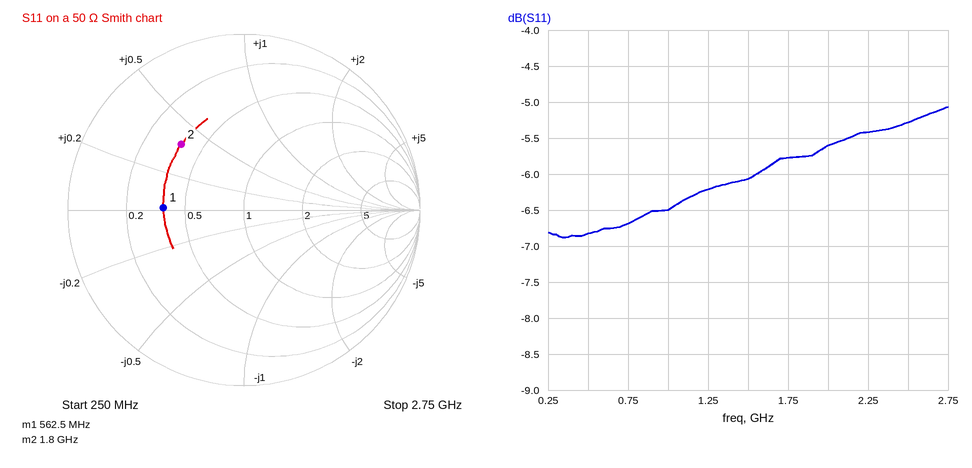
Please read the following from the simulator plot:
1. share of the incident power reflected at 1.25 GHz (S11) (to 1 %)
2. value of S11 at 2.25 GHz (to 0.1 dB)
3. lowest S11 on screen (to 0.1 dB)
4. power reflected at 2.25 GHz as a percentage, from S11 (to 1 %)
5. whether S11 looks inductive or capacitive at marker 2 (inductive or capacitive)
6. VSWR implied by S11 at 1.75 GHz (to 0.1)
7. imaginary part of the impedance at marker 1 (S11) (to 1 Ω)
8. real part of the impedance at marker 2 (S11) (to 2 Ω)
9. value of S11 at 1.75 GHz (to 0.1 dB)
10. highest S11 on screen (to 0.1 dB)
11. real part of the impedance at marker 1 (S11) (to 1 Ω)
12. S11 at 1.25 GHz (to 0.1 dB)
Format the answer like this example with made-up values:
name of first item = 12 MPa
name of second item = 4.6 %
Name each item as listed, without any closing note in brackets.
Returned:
share of the incident power reflected at 1.25 GHz (S11) = 24 %
value of S11 at 2.25 GHz = -5.4 dB
lowest S11 on screen = -6.9 dB
power reflected at 2.25 GHz as a percentage, from S11 = 29 %
whether S11 looks inductive or capacitive at marker 2 = inductive
VSWR implied by S11 at 1.75 GHz = 3.1
imaginary part of the impedance at marker 1 (S11) = +1 Ω
real part of the impedance at marker 2 (S11) = 18 Ω
value of S11 at 1.75 GHz = -5.8 dB
highest S11 on screen = -5.1 dB
real part of the impedance at marker 1 (S11) = 19 Ω
S11 at 1.25 GHz = -6.2 dB
